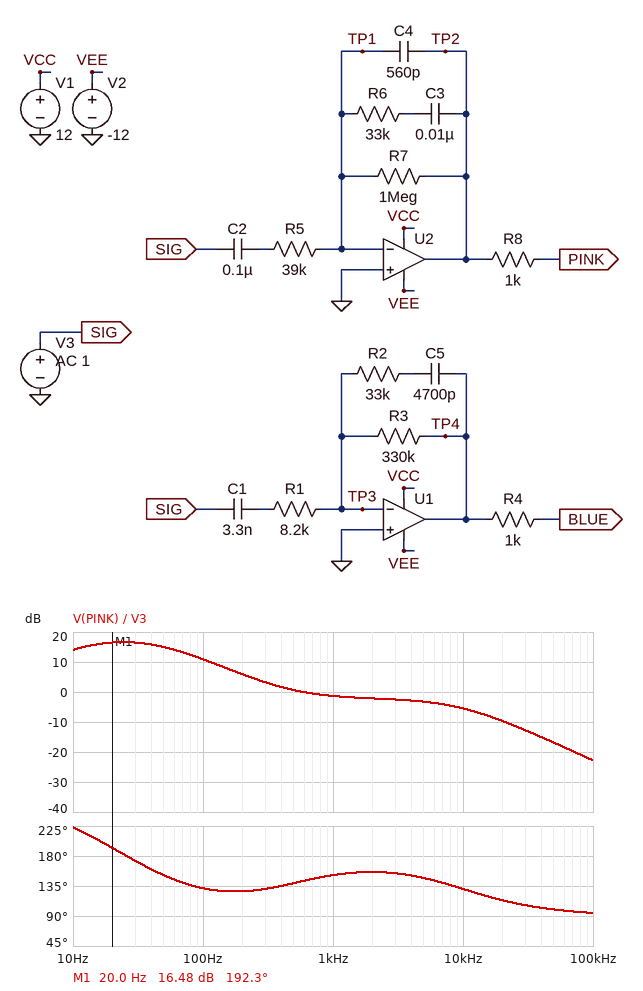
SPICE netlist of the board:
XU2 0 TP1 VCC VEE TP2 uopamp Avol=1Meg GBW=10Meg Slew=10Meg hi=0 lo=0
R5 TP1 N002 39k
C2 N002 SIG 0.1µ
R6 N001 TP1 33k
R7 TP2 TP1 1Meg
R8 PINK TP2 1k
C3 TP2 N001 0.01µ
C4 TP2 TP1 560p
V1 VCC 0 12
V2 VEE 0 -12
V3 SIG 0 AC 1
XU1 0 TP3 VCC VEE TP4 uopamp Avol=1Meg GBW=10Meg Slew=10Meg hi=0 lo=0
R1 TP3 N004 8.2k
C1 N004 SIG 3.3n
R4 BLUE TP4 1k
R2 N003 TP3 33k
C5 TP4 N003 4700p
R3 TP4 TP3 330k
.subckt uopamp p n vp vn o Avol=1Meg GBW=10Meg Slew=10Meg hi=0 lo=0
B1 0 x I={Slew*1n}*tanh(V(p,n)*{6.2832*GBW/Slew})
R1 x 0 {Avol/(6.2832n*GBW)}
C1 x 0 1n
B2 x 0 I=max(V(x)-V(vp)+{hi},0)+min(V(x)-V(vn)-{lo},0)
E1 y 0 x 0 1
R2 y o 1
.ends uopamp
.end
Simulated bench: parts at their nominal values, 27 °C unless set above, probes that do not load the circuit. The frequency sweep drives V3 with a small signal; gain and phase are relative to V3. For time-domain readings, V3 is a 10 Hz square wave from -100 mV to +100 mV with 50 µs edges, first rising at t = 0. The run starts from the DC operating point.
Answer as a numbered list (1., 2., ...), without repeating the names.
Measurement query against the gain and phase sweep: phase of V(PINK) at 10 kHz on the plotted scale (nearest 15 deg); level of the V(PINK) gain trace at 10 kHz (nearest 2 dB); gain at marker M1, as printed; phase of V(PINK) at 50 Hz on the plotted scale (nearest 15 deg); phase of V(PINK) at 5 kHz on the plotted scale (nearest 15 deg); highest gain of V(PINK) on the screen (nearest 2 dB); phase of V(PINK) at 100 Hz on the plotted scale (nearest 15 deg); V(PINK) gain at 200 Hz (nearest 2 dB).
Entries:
1. 135 deg
2. -6 dB
3. 16.48 dB
4. 150 deg
5. 150 deg
6. 16 dB
7. 135 deg
8. 6 dB
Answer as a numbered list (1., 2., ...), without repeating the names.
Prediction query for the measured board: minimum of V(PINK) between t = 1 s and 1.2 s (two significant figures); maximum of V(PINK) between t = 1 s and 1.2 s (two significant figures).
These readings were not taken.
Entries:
1. -1.0 V
2. 1.0 V
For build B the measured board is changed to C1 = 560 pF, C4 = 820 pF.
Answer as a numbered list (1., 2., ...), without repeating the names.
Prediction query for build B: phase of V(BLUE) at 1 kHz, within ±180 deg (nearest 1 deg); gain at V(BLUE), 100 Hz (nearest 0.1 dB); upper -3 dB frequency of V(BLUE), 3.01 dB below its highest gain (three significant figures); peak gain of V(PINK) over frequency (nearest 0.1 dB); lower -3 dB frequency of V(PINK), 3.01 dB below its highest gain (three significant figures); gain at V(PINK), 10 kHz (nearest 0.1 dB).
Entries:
1. -132 deg
2. -22.0 dB
3. 2.19 MHz
4. 16.5 dB
5. 9.11 Hz
6. -7.6 dB
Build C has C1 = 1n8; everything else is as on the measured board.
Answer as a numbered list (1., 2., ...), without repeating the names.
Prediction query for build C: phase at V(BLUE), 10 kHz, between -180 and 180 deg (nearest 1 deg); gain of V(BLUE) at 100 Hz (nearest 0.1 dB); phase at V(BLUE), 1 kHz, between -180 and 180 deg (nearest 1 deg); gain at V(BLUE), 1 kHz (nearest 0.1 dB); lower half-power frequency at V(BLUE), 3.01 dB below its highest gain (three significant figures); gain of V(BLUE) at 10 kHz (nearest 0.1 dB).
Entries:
1. -138 deg
2. -11.8 dB
3. -136 deg
4. -6.3 dB
5. 10.6 kHz
6. 8.0 dB
